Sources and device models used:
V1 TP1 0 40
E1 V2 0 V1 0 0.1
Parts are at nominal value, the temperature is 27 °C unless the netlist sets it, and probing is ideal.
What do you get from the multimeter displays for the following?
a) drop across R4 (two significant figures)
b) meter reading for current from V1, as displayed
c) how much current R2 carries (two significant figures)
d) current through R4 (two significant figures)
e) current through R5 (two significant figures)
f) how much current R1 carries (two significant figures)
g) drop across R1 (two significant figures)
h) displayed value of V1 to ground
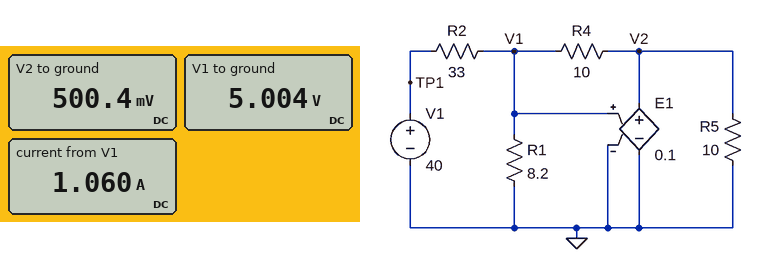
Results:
4.5 V
1.060 A
1.1 A
450 mA
50 mA
610 mA
5.0 V
5.004 V
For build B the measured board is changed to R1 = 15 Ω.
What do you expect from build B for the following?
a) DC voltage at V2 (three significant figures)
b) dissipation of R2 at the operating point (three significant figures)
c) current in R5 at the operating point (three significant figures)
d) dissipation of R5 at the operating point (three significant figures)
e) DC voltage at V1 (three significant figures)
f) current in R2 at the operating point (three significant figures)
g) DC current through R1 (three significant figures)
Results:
648 mV
34.0 W
64.8 mA
42.0 mW
6.48 V
1.02 A
432 mA
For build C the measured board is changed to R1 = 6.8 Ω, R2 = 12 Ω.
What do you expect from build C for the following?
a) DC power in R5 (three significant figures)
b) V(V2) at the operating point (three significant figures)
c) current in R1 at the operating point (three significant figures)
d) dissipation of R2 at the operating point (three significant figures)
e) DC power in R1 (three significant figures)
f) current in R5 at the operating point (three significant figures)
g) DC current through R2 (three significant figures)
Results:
108 mW
1.04 V
1.53 A
73.0 W
15.9 W
104 mA
2.47 A
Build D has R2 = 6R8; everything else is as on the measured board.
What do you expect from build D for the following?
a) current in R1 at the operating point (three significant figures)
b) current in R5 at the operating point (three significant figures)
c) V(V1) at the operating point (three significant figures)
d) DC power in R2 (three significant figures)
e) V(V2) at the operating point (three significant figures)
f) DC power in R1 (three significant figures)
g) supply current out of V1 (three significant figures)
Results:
2.00 A
164 mA
16.4 V
82.0 W
1.64 V
32.7 W
3.47 A
